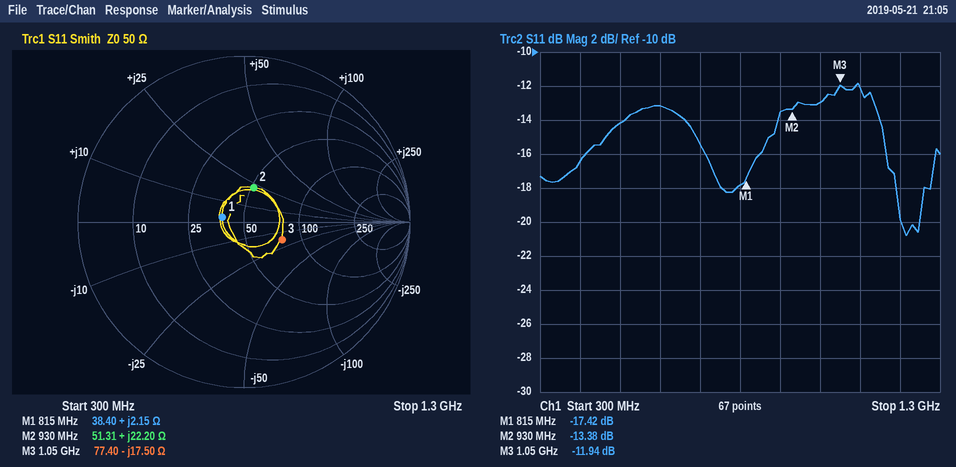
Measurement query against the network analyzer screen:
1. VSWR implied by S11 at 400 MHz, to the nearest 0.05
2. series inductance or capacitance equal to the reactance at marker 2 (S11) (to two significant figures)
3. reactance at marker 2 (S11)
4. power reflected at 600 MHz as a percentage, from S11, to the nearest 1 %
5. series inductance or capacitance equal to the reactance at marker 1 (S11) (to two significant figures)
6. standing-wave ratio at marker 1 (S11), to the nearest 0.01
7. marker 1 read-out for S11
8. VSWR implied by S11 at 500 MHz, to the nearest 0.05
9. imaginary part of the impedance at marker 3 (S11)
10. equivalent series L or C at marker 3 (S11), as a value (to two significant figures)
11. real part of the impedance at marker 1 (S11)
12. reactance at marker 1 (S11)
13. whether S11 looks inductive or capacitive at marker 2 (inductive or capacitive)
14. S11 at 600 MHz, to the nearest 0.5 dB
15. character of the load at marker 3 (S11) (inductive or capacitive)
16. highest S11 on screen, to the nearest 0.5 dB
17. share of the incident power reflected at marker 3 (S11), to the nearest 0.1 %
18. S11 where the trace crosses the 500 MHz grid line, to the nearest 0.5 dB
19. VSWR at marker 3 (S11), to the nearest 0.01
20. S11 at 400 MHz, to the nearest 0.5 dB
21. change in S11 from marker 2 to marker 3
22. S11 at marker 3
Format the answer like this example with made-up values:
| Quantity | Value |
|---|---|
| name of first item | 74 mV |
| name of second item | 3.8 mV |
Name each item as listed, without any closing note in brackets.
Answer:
| Quantity | Value |
|---|---|
| VSWR implied by S11 at 400 MHz, to the nearest 0.05 | 1.35 |
| series inductance or capacitance equal to the reactance at marker 2 (S11) | 3.8 nH |
| reactance at marker 2 | +22.20 Ω |
| power reflected at 600 MHz as a percentage, from S11, to the nearest 1 % | 5 % |
| series inductance or capacitance equal to the reactance at marker 1 (S11) | 420 pH |
| standing-wave ratio at marker 1 (S11), to the nearest 0.01 | 1.31 |
| marker 1 read-out for S11 | -17.42 dB |
| VSWR implied by S11 at 500 MHz, to the nearest 0.05 | 1.50 |
| imaginary part of the impedance at marker 3 | -17.50 Ω |
| equivalent series L or C at marker 3 (S11), as a value | 8.7 pF |
| real part of the impedance at marker 1 | 38.40 Ω |
| reactance at marker 1 | +2.15 Ω |
| whether S11 looks inductive or capacitive at marker 2 | inductive |
| S11 at 600 MHz, to the nearest 0.5 dB | -13.0 dB |
| character of the load at marker 3 (S11) | capacitive |
| highest S11 on screen, to the nearest 0.5 dB | -12.0 dB |
| share of the incident power reflected at marker 3 (S11), to the nearest 0.1 % | 6.4 % |
| S11 where the trace crosses the 500 MHz grid line, to the nearest 0.5 dB | -14.0 dB |
| VSWR at marker 3 (S11), to the nearest 0.01 | 1.68 |
| S11 at 400 MHz, to the nearest 0.5 dB | -16.5 dB |
| change in S11 from marker 2 to marker 3 | 1.44 dB |
| S11 at marker 3 | -11.94 dB |
